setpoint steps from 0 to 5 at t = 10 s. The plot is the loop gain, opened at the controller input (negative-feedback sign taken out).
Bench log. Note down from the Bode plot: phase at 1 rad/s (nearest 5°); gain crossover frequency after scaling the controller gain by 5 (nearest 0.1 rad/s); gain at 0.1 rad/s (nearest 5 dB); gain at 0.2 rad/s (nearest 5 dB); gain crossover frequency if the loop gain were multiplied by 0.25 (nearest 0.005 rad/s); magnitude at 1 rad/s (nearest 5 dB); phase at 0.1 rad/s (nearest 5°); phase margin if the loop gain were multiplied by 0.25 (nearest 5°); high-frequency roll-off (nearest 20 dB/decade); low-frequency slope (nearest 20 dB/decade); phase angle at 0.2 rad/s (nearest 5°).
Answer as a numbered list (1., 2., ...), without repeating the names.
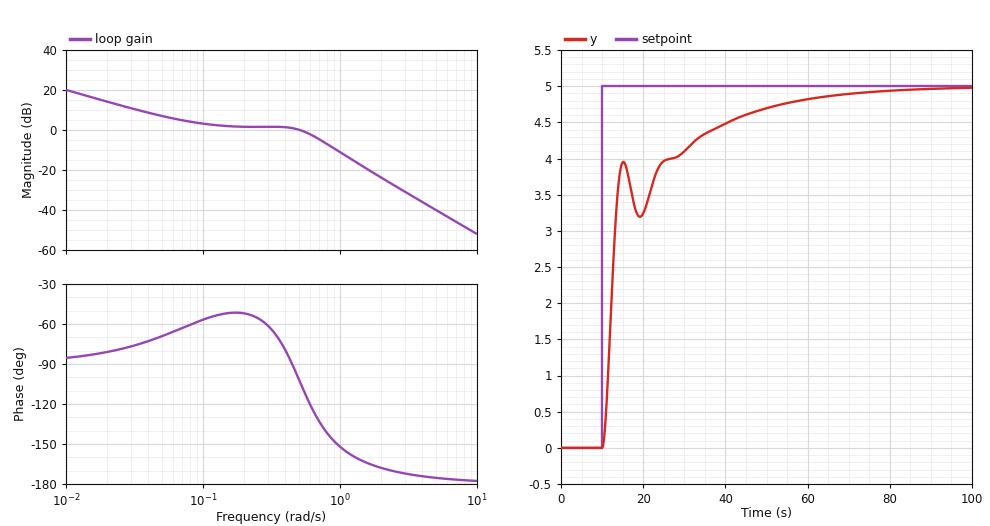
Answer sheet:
1. -150°
2. 1.2 rad/s
3. 5 dB
4. 0 dB
5. 0.025 rad/s
6. -10 dB
7. -55°
8. 100°
9. -40 dB/decade
10. -20 dB/decade
11. -50°
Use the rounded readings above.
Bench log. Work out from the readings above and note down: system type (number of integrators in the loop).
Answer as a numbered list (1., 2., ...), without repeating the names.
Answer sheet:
1. 1
